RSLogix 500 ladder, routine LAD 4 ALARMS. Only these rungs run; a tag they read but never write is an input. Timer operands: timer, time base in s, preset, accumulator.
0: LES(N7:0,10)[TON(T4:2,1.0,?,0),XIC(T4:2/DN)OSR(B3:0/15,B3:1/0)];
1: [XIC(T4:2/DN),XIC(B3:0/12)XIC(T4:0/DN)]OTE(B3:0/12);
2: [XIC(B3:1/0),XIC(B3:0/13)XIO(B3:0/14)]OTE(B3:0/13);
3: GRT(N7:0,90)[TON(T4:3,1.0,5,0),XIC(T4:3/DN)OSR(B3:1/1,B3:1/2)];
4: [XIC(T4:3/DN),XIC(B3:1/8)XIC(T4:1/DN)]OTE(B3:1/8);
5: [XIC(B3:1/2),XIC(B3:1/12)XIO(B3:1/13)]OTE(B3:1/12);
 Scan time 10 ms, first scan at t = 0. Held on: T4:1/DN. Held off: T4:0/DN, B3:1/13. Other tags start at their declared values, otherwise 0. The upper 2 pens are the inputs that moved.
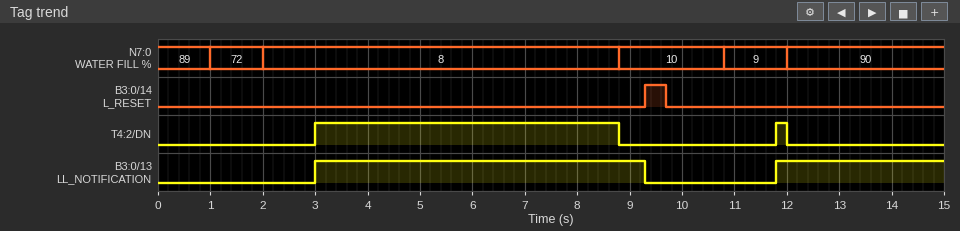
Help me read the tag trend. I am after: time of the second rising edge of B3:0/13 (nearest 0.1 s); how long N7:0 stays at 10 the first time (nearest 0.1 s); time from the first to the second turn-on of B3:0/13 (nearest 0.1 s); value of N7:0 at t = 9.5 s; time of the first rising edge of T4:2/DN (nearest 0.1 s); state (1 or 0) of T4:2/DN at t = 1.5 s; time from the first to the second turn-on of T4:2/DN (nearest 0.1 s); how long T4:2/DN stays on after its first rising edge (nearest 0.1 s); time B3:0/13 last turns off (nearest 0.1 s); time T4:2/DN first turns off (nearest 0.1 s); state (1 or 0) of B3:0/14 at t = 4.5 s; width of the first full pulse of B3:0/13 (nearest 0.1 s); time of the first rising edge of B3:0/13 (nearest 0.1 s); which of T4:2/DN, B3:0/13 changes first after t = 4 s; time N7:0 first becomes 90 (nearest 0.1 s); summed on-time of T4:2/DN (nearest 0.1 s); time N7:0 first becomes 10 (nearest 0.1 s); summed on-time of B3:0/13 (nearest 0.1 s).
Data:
11.8 s
2.0 s
8.8 s
10
3.0 s
0
8.8 s
5.8 s
9.3 s
8.8 s
0
6.3 s
3.0 s
T4:2/DN
12.0 s
6.0 s
8.8 s
9.5 s
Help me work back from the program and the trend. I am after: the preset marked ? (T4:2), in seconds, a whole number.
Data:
1 s
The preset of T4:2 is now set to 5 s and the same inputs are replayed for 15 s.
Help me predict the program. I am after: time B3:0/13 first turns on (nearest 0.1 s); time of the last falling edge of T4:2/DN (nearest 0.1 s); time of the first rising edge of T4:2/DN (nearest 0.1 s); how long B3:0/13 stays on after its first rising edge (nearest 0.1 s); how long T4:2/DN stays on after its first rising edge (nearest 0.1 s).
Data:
7.0 s
8.8 s
7.0 s
2.3 s
1.8 s
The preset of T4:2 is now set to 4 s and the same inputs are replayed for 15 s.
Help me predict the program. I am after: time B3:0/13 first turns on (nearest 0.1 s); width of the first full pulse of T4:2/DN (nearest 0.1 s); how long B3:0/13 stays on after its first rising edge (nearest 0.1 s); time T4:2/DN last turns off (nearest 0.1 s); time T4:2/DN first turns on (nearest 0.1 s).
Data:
6.0 s
2.8 s
3.3 s
8.8 s
6.0 s
